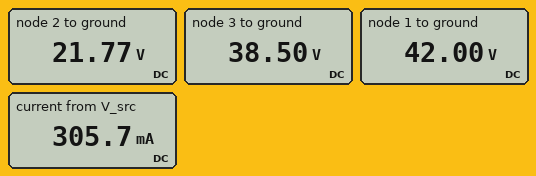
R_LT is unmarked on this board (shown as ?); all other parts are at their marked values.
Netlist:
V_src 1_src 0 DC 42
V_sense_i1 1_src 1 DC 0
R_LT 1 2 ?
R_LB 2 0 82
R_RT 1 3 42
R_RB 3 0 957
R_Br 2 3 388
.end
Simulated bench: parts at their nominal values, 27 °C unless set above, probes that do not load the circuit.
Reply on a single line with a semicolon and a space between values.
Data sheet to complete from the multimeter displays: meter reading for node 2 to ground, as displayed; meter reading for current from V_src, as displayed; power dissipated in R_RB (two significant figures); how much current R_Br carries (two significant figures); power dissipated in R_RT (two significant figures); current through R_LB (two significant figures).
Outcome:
21.77 V; 305.7 mA; 1.5 W; 43 mA; 290 mW; 270 mA
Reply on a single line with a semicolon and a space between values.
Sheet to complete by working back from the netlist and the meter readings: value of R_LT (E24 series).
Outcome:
91 Ω
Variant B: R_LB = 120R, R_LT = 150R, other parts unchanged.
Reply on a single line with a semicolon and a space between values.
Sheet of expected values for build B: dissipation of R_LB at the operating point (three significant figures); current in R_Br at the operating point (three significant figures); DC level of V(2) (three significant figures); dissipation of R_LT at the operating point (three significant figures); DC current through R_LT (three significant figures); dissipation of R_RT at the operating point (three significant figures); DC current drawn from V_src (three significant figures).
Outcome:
3.88 W; 43.6 mA; 21.6 V; 2.78 W; 136 mA; 295 mW; 220 mA
